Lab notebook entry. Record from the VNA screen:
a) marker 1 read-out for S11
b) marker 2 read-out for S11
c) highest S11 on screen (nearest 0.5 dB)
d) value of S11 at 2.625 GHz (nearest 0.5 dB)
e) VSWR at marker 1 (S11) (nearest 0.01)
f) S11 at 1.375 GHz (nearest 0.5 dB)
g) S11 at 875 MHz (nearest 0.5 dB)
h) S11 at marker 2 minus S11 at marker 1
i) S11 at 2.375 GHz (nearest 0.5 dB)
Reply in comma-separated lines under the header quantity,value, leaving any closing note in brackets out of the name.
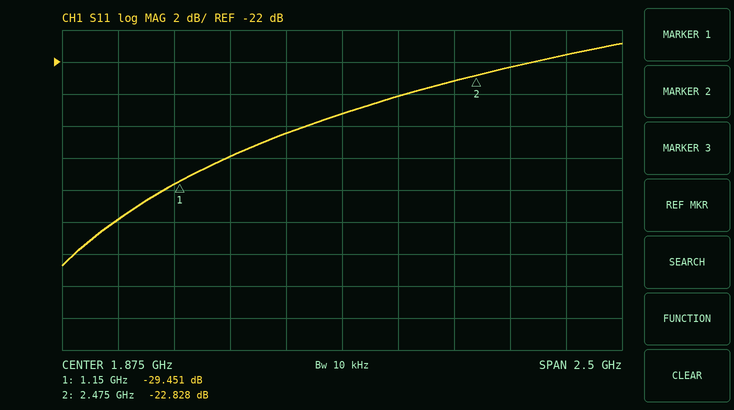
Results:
quantity,value
marker 1 read-out for S11,-29.451 dB
marker 2 read-out for S11,-22.828 dB
highest S11 on screen,-21.0 dB
value of S11 at 2.625 GHz,-22.5 dB
VSWR at marker 1 (S11),1.07
S11 at 1.375 GHz,-28.0 dB
S11 at 875 MHz,-32.0 dB
S11 at marker 2 minus S11 at marker 1,6.623 dB
S11 at 2.375 GHz,-23.0 dB
